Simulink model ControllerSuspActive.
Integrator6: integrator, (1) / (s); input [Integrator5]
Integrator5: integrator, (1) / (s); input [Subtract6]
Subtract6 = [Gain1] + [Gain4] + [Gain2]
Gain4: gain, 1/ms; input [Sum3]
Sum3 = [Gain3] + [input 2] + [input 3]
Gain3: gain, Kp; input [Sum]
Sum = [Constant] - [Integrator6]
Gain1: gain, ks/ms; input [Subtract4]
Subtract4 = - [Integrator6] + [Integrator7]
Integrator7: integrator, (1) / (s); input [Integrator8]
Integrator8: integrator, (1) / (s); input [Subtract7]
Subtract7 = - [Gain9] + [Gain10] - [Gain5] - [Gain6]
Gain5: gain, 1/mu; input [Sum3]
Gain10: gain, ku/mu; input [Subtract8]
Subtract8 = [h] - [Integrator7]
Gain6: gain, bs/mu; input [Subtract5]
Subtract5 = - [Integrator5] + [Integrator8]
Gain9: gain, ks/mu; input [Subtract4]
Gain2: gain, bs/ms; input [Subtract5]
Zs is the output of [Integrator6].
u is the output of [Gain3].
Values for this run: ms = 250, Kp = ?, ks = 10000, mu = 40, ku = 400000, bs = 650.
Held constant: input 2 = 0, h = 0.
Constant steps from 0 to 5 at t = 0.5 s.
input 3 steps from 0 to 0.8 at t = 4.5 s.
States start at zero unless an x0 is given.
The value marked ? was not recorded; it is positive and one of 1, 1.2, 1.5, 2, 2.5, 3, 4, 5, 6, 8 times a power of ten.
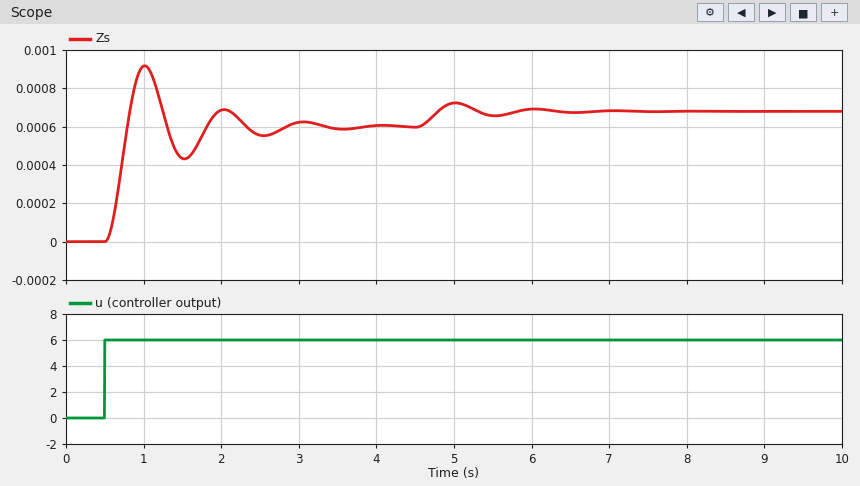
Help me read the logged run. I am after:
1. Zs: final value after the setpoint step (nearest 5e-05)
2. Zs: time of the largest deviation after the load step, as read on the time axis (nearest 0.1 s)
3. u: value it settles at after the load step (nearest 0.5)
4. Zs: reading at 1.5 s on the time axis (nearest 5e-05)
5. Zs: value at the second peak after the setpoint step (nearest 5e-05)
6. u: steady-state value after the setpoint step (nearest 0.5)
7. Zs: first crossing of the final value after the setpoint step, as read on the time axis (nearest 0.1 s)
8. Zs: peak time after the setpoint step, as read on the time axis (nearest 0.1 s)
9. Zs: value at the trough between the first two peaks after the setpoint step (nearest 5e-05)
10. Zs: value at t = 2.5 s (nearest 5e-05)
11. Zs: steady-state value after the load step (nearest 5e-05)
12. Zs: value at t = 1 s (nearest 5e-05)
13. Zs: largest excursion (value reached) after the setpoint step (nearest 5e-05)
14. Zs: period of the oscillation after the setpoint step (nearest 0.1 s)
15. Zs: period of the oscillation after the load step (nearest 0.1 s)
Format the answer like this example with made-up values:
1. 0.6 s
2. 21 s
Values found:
1. 0.00060
2. 5.0 s
3. 6.0
4. 0.00045
5. 0.00070
6. 6.0
7. 0.8 s
8. 1.0 s
9. 0.00045
10. 0.00055
11. 0.00070
12. 0.00090
13. 0.00090
14. 1.0 s
15. 1.0 s
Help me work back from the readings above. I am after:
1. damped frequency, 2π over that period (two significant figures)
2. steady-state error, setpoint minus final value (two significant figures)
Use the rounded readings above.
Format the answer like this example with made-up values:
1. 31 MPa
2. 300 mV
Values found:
1. 6.3 rad/s
2. 5.0
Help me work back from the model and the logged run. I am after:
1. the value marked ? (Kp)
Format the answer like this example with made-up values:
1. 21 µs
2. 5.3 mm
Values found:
1. 1.2
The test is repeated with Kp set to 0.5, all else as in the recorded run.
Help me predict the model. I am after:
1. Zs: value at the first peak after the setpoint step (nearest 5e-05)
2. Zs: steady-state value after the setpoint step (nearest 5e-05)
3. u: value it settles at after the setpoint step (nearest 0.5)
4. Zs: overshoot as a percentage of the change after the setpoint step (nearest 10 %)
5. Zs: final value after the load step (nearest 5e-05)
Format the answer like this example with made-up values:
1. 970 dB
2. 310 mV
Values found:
1. 0.00040
2. 0.00025
3. 2.5
4. 50 %
5. 0.00035
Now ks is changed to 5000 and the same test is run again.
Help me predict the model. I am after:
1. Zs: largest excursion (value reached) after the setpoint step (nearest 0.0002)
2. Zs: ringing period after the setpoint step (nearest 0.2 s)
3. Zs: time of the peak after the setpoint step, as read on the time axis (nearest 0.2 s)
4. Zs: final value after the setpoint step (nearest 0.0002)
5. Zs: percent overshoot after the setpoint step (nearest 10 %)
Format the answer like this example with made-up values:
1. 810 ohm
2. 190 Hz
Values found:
1. 0.0016
2. 1.4 s
3. 1.2 s
4. 0.0012
5. 40 %
